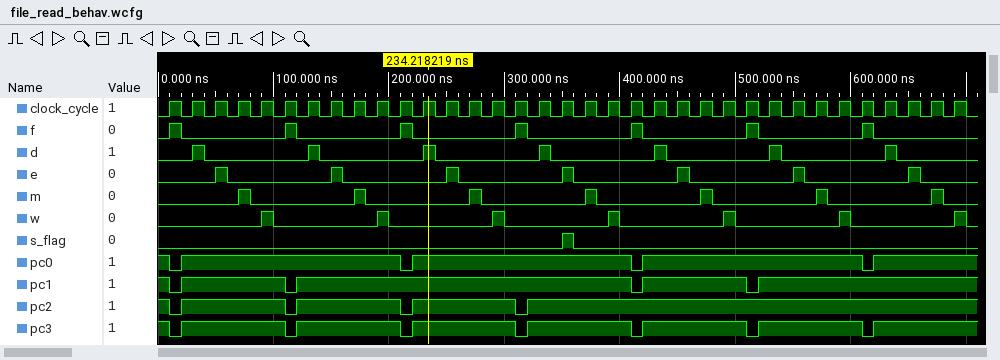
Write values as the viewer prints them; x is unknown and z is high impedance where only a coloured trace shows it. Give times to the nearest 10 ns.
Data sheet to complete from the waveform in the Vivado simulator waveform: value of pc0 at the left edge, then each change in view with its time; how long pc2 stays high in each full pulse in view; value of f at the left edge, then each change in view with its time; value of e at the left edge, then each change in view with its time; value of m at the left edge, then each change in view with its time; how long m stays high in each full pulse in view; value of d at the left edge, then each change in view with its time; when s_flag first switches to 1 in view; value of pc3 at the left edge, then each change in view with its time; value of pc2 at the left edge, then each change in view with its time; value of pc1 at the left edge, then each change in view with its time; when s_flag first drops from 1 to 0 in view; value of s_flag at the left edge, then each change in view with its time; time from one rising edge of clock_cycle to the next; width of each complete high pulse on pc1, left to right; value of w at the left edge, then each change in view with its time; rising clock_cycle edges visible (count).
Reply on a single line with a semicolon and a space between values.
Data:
1, 0 at 10 ns, 1 at 20 ns, 0 at 210 ns, 1 at 220 ns, 0 at 410 ns, 1 at 420 ns, 0 at 610 ns, 1 at 620 ns; 90 ns, 90 ns, 90 ns; 0, 1 at 10 ns, 0 at 20 ns, 1 at 110 ns, 0 at 120 ns, 1 at 210 ns, 0 at 220 ns, 1 at 310 ns, 0 at 320 ns, 1 at 410 ns, 0 at 420 ns, 1 at 510 ns, 0 at 520 ns, 1 at 610 ns, 0 at 620 ns; 0, 1 at 50 ns, 0 at 60 ns, 1 at 150 ns, 0 at 160 ns, 1 at 250 ns, 0 at 260 ns, 1 at 350 ns, 0 at 360 ns, 1 at 450 ns, 0 at 460 ns, 1 at 550 ns, 0 at 560 ns, 1 at 650 ns, 0 at 660 ns; 0, 1 at 70 ns, 0 at 80 ns, 1 at 170 ns, 0 at 180 ns, 1 at 270 ns, 0 at 280 ns, 1 at 370 ns, 0 at 380 ns, 1 at 470 ns, 0 at 480 ns, 1 at 570 ns, 0 at 580 ns, 1 at 670 ns, 0 at 680 ns; 10 ns, 10 ns, 10 ns, 10 ns, 10 ns, 10 ns, 10 ns; 0, 1 at 30 ns, 0 at 40 ns, 1 at 130 ns, 0 at 140 ns, 1 at 230 ns, 0 at 240 ns, 1 at 330 ns, 0 at 340 ns, 1 at 430 ns, 0 at 440 ns, 1 at 530 ns, 0 at 540 ns, 1 at 630 ns, 0 at 640 ns; 350 ns; 1, 0 at 10 ns, 1 at 20 ns, 0 at 110 ns, 1 at 120 ns, 0 at 210 ns, 1 at 220 ns, 0 at 310 ns, 1 at 320 ns, 0 at 410 ns, 1 at 420 ns, 0 at 510 ns, 1 at 520 ns, 0 at 610 ns, 1 at 620 ns; 1, 0 at 10 ns, 1 at 20 ns, 0 at 110 ns, 1 at 120 ns, 0 at 210 ns, 1 at 220 ns, 0 at 310 ns, 1 at 320 ns; 1, 0 at 10 ns, 1 at 20 ns, 0 at 110 ns, 1 at 120 ns, 0 at 410 ns, 1 at 420 ns, 0 at 510 ns, 1 at 520 ns; 360 ns; 0, 1 at 350 ns, 0 at 360 ns; 20 ns; 90 ns, 290 ns, 90 ns; 0, 1 at 90 ns, 0 at 100 ns, 1 at 190 ns, 0 at 200 ns, 1 at 290 ns, 0 at 300 ns, 1 at 390 ns, 0 at 400 ns, 1 at 490 ns, 0 at 500 ns, 1 at 590 ns, 0 at 600 ns, 1 at 690 ns, 0 at 700 ns; 35
